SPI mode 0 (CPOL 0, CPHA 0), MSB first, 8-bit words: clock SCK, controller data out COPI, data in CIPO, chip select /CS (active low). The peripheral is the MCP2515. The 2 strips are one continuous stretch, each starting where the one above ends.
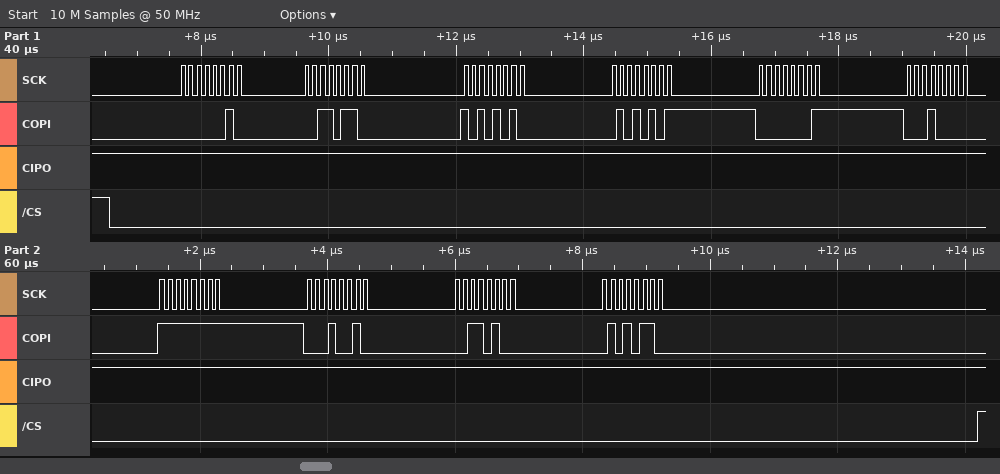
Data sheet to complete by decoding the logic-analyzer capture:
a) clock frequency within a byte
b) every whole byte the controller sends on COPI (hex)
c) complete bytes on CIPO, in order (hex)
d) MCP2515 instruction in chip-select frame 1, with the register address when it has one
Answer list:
8 MHz
02 36 AA 55 01 10 FF 12 34 56
FF FF FF FF FF FF FF FF FF FF
WRITE 0x36
